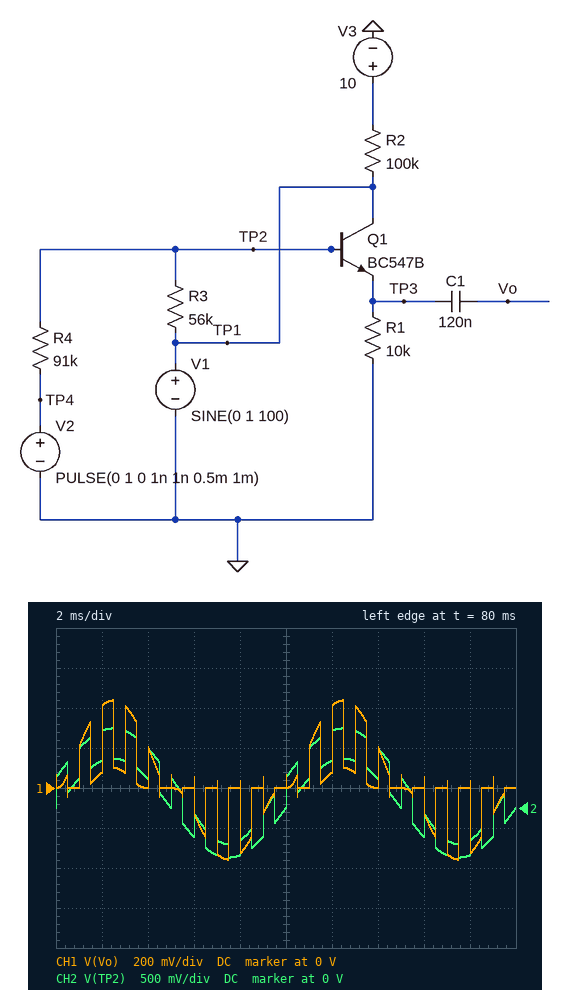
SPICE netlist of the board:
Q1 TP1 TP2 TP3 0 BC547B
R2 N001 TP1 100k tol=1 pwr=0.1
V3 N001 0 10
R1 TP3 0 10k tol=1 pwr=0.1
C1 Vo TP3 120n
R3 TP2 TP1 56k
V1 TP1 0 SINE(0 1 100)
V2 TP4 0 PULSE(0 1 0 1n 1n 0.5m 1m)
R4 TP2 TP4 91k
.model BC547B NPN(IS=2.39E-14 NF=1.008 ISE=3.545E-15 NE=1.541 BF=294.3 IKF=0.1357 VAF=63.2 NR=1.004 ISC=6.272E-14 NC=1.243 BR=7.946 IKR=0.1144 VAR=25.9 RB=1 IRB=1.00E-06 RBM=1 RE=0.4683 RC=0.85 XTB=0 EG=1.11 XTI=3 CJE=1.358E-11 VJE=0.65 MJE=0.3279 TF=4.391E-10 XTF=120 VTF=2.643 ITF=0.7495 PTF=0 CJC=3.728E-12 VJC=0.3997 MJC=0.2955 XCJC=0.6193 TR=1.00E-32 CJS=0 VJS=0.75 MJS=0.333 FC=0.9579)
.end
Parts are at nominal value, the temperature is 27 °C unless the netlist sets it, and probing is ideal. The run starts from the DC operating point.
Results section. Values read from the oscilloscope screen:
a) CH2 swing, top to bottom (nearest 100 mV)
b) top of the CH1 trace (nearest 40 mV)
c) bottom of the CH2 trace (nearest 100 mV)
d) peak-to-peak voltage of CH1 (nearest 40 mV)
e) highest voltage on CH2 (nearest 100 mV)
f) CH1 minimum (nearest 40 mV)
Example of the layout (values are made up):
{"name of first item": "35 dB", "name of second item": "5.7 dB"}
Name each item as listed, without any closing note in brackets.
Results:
{"CH2 swing, top to bottom": "1.6 V", "top of the CH1 trace": "440 mV", "bottom of the CH2 trace": "-600 mV", "peak-to-peak voltage of CH1": "800 mV", "highest voltage on CH2": "1.0 V", "CH1 minimum": "-360 mV"}
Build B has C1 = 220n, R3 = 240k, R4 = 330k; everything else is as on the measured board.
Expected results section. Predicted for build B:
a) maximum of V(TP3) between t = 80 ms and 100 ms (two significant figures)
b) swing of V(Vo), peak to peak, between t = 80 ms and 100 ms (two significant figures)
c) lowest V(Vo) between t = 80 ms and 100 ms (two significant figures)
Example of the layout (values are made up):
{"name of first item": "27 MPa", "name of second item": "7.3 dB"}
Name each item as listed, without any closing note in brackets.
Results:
{"maximum of V(TP3) between t = 80 ms and 100 ms": "420 mV", "swing of V(Vo), peak to peak, between t = 80 ms and 100 ms": "550 mV", "lowest V(Vo) between t = 80 ms and 100 ms": "-130 mV"}
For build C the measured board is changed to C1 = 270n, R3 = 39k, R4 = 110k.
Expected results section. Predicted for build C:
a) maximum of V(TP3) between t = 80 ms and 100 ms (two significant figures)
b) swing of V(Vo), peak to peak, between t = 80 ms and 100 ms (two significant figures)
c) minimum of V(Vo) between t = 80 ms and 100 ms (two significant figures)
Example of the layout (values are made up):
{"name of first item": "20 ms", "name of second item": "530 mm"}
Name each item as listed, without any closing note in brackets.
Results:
{"maximum of V(TP3) between t = 80 ms and 100 ms": "440 mV", "swing of V(Vo), peak to peak, between t = 80 ms and 100 ms": "490 mV", "minimum of V(Vo) between t = 80 ms and 100 ms": "-55 mV"}
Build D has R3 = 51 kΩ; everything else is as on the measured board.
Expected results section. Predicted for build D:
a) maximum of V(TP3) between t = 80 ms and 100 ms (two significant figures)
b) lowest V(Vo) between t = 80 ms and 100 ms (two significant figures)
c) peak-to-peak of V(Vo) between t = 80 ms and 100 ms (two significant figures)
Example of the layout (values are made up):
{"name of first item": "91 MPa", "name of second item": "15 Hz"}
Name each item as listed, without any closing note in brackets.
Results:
{"maximum of V(TP3) between t = 80 ms and 100 ms": "440 mV", "lowest V(Vo) between t = 80 ms and 100 ms": "-310 mV", "peak-to-peak of V(Vo) between t = 80 ms and 100 ms": "750 mV"}
